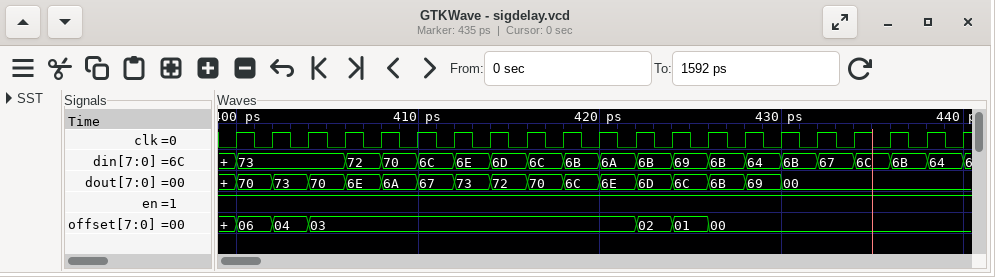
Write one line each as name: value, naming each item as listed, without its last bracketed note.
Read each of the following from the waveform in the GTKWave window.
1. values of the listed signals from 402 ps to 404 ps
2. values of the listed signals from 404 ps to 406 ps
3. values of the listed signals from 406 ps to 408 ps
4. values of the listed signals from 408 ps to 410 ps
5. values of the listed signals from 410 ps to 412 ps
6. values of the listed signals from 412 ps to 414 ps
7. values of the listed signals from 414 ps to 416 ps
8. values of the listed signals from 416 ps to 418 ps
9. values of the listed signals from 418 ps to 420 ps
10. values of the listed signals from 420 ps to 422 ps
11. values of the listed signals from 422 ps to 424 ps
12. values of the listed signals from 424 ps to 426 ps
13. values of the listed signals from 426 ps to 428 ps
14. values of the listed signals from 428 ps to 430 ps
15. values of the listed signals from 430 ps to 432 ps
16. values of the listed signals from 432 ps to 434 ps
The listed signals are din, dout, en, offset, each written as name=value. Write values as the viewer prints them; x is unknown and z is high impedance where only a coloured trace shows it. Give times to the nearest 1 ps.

values of the listed signals from 402 ps to 404 ps: din=73, dout=73, en=1, offset=04
values of the listed signals from 404 ps to 406 ps: din=73, dout=70, en=1, offset=03
values of the listed signals from 406 ps to 408 ps: din=72, dout=6E, en=1, offset=03
values of the listed signals from 408 ps to 410 ps: din=70, dout=6A, en=1, offset=03
values of the listed signals from 410 ps to 412 ps: din=6C, dout=67, en=1, offset=03
values of the listed signals from 412 ps to 414 ps: din=6E, dout=73, en=1, offset=03
values of the listed signals from 414 ps to 416 ps: din=6D, dout=72, en=1, offset=03
values of the listed signals from 416 ps to 418 ps: din=6C, dout=70, en=1, offset=03
values of the listed signals from 418 ps to 420 ps: din=6B, dout=6C, en=1, offset=03
values of the listed signals from 420 ps to 422 ps: din=6A, dout=6E, en=1, offset=03
values of the listed signals from 422 ps to 424 ps: din=6B, dout=6D, en=1, offset=02
values of the listed signals from 424 ps to 426 ps: din=69, dout=6C, en=1, offset=01
values of the listed signals from 426 ps to 428 ps: din=6B, dout=6B, en=1, offset=00
values of the listed signals from 428 ps to 430 ps: din=64, dout=69, en=1, offset=00
values of the listed signals from 430 ps to 432 ps: din=6B, dout=00, en=1, offset=00
values of the listed signals from 432 ps to 434 ps: din=67, dout=00, en=1, offset=00
